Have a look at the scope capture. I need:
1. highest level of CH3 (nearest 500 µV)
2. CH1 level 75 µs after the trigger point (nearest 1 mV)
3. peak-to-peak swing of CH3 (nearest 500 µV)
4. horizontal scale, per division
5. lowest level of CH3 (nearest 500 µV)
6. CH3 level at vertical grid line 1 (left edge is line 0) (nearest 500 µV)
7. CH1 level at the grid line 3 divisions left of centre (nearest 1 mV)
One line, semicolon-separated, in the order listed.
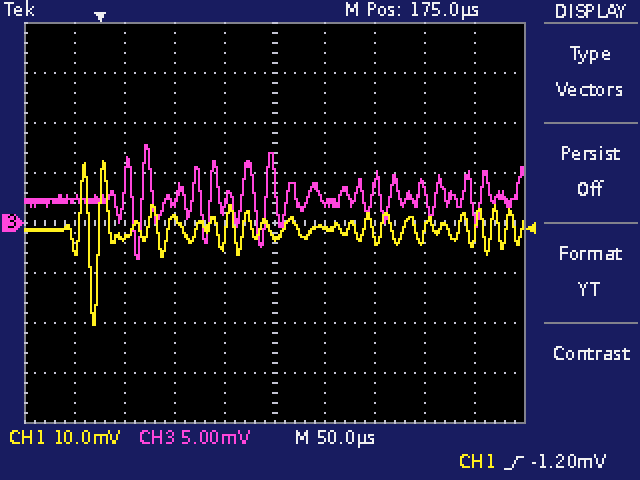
8.0 mV; 1 mV; 11.5 mV; 50 µs; -3.5 mV; 2.5 mV; -3 mV
